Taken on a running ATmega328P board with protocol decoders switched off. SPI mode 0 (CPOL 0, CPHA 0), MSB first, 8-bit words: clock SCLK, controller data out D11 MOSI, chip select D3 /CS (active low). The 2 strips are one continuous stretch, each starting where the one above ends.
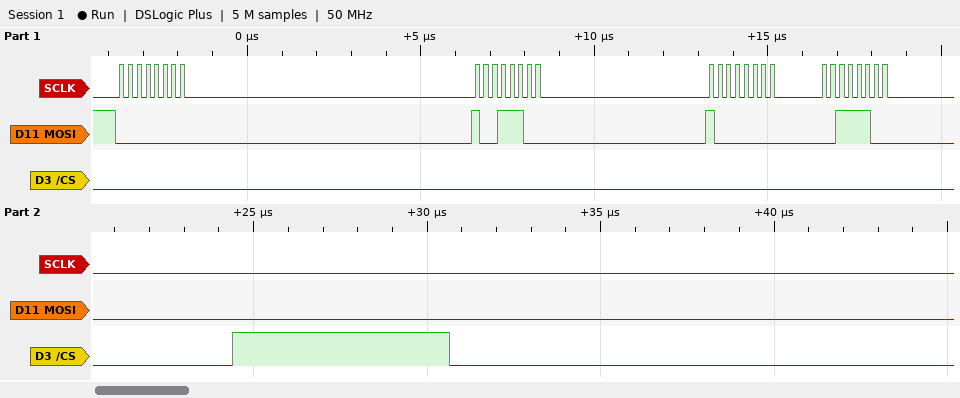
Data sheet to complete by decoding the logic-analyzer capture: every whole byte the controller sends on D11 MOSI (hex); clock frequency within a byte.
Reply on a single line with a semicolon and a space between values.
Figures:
00 9C 80 3C; 4 MHz
